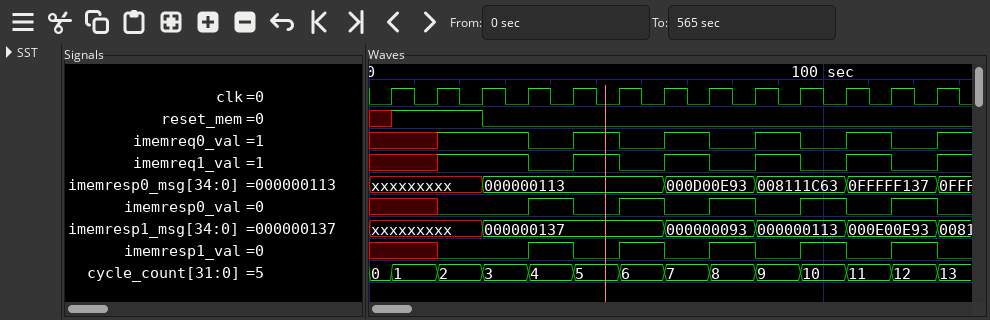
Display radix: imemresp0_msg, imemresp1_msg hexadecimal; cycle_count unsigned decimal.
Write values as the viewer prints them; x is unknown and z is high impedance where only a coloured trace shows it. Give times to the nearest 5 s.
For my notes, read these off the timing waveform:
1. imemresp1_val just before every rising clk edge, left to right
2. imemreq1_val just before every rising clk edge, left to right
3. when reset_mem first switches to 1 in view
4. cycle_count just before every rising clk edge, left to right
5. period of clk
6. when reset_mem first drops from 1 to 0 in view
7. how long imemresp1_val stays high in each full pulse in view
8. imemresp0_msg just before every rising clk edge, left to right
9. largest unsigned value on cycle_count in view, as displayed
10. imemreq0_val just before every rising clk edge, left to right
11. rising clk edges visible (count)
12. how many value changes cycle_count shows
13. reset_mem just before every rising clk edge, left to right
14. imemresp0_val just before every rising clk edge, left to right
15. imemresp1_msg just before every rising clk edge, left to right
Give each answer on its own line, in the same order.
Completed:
x x 0 0 1 0 1 0 1 0 1 0 1
x x 1 1 0 1 0 1 0 1 0 1 0
5 s
0, 1, 2, 3, 4, 5, 6, 7, 8, 9, 10, 11, 12
10 s
25 s
10 s, 10 s, 10 s, 10 s, 10 s
xxxxxxxxx, xxxxxxxxx, xxxxxxxxx, 000000113, 000000113, 000000113, 000000113, 000D00E93, 000D00E93, 008111C63, 008111C63, 0FFFFF137, 0FFFFF137
13
x x 1 1 0 1 0 1 0 1 0 1 0
13
13
x 1 1 0 0 0 0 0 0 0 0 0 0
x x 0 0 1 0 1 0 1 0 1 0 1
xxxxxxxxx, xxxxxxxxx, xxxxxxxxx, 000000137, 000000137, 000000137, 000000137, 000000093, 000000093, 000000113, 000000113, 000E00E93, 000E00E93
